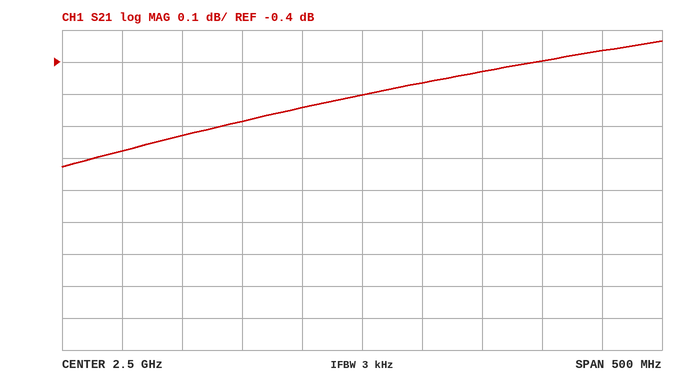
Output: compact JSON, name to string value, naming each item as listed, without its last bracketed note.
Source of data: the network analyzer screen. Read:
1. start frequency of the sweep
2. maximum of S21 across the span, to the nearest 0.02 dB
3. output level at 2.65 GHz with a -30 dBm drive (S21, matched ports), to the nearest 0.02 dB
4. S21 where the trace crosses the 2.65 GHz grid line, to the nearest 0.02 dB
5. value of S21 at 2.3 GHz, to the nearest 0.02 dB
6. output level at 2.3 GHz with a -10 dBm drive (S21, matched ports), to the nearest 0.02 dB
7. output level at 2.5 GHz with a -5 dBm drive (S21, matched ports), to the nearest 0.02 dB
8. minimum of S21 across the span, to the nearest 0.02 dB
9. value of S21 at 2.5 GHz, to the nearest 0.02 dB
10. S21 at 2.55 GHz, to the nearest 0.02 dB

{"start frequency of the sweep": "2.25 GHz", "maximum of S21 across the span, to the nearest 0.02 dB": "-0.34 dB", "output level at 2.65 GHz with a -30 dBm drive (S21, matched ports), to the nearest 0.02 dB": "-30.40 dBm", "S21 where the trace crosses the 2.65 GHz grid line, to the nearest 0.02 dB": "-0.40 dB", "value of S21 at 2.3 GHz, to the nearest 0.02 dB": "-0.68 dB", "output level at 2.3 GHz with a -10 dBm drive (S21, matched ports), to the nearest 0.02 dB": "-10.68 dBm", "output level at 2.5 GHz with a -5 dBm drive (S21, matched ports), to the nearest 0.02 dB": "-5.50 dBm", "minimum of S21 across the span, to the nearest 0.02 dB": "-0.72 dB", "value of S21 at 2.5 GHz, to the nearest 0.02 dB": "-0.50 dB", "S21 at 2.55 GHz, to the nearest 0.02 dB": "-0.46 dB"}
